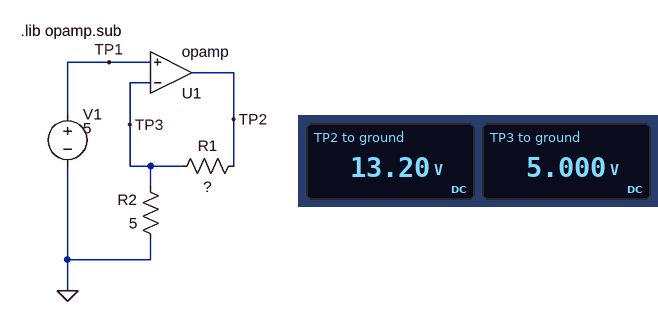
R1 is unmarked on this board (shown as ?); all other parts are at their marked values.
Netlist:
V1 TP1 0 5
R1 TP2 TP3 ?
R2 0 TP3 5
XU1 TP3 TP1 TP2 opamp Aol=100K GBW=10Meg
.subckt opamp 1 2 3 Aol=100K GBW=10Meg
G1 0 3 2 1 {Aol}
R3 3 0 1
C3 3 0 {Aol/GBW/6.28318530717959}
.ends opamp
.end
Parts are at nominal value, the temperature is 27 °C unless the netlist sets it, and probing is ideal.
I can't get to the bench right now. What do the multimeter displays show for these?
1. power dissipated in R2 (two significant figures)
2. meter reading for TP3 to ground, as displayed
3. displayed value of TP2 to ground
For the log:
5.0 W
5.000 V
13.20 V
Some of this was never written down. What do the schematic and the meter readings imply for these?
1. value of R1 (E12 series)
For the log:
8.2 Ω
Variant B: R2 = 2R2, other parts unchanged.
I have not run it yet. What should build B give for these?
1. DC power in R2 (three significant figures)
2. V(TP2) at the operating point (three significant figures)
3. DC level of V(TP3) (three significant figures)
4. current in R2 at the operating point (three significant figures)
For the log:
11.4 W
23.6 V
5.00 V
2.27 A
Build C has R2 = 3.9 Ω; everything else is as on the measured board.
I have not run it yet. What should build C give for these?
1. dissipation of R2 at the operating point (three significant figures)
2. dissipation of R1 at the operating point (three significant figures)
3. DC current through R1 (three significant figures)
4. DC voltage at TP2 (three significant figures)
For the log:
6.41 W
13.5 W
1.28 A
15.5 V
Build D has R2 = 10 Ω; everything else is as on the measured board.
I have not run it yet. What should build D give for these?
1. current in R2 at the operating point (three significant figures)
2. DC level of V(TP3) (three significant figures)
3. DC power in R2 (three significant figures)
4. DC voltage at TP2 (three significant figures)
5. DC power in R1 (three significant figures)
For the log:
500 mA
5.00 V
2.50 W
9.10 V
2.05 W
